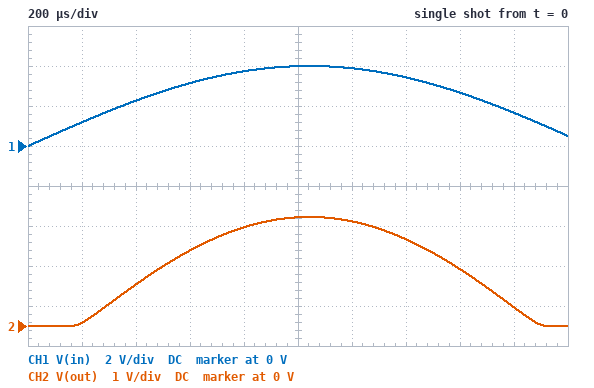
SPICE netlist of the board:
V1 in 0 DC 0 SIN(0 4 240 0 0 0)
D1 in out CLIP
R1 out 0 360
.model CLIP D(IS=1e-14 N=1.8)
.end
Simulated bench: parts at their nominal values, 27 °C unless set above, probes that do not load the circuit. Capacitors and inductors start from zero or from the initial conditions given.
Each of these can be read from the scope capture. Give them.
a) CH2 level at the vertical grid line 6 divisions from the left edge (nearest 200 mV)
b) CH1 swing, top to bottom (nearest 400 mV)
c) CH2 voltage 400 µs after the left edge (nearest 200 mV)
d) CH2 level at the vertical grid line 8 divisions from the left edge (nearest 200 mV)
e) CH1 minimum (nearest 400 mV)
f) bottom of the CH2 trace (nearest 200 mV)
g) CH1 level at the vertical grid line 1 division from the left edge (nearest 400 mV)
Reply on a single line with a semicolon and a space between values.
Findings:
2.6 V; 4.0 V; 1.0 V; 1.4 V; 0 V; 0 V; 1.2 V
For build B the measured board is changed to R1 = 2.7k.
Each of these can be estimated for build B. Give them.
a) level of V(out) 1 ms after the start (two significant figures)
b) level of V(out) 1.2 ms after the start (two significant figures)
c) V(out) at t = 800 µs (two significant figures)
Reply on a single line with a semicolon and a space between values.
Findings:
2.8 V; 2.7 V; 2.6 V
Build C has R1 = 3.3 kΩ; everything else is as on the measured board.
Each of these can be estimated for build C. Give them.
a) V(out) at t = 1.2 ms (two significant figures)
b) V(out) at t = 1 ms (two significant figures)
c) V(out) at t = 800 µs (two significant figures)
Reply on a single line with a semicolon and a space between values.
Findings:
2.7 V; 2.8 V; 2.6 V
